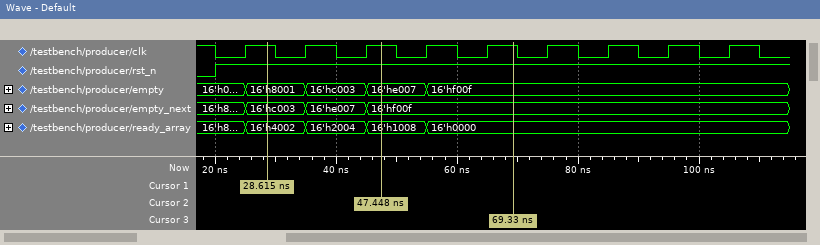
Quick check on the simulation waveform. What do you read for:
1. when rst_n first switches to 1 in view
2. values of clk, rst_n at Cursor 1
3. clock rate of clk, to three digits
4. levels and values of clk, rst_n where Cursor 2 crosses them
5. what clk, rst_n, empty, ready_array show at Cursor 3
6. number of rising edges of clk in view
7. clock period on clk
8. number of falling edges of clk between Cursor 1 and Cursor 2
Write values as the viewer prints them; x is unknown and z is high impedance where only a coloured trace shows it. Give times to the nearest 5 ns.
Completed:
20 ns
clk=1, rst_n=1
100 MHz
clk=1, rst_n=1
clk=1, rst_n=1, empty=16'hf00f, ready_array=16'h0000
9
10 ns
2
